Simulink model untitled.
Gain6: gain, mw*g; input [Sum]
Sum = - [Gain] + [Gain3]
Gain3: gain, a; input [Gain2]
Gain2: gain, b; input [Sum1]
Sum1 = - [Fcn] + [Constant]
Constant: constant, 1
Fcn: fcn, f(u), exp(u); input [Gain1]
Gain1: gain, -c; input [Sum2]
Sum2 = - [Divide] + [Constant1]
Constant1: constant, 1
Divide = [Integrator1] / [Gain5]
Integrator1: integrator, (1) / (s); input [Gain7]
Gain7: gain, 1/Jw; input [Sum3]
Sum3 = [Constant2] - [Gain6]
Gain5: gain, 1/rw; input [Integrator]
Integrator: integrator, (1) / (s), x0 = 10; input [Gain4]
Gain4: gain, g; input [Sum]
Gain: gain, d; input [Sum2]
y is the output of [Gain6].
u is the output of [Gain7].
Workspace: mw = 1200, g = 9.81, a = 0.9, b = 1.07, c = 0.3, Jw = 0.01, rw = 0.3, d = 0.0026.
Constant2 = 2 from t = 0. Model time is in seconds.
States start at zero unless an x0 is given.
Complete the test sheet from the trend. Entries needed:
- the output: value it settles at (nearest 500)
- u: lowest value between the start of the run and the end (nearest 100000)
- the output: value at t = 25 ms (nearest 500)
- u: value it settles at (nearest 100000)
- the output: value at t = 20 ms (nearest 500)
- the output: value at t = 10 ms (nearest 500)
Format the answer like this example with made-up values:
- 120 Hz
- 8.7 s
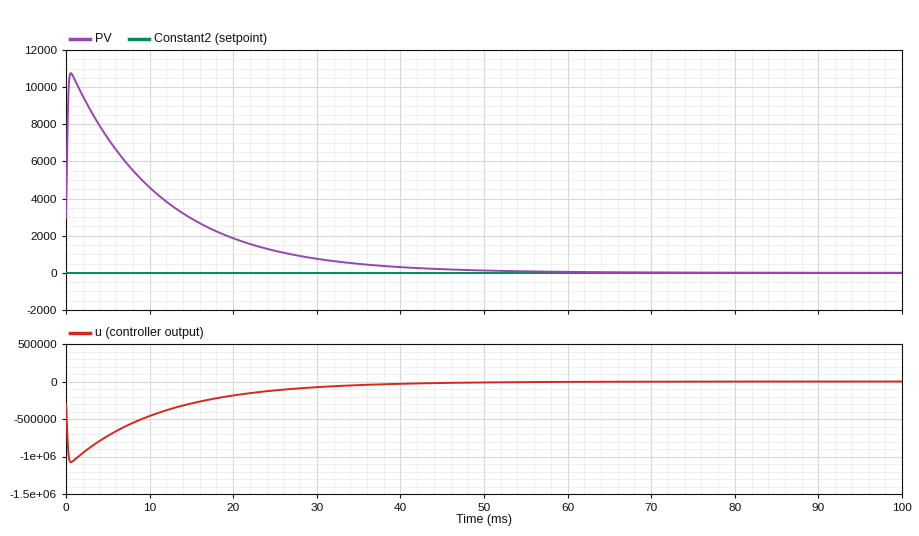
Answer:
- 0
- -1100000
- 1000
- 0
- 2000
- 4500
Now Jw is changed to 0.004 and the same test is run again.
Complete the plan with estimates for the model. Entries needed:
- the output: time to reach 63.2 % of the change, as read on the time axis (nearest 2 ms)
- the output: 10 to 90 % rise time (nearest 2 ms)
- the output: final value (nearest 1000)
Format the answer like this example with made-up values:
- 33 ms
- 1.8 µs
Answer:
- 10 ms
- 10 ms
- 0
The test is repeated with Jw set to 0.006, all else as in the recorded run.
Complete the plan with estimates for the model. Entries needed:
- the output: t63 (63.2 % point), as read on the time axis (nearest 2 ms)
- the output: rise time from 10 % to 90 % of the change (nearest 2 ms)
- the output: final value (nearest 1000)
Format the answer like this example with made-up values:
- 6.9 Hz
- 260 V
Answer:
- 16 ms
- 14 ms
- 0
